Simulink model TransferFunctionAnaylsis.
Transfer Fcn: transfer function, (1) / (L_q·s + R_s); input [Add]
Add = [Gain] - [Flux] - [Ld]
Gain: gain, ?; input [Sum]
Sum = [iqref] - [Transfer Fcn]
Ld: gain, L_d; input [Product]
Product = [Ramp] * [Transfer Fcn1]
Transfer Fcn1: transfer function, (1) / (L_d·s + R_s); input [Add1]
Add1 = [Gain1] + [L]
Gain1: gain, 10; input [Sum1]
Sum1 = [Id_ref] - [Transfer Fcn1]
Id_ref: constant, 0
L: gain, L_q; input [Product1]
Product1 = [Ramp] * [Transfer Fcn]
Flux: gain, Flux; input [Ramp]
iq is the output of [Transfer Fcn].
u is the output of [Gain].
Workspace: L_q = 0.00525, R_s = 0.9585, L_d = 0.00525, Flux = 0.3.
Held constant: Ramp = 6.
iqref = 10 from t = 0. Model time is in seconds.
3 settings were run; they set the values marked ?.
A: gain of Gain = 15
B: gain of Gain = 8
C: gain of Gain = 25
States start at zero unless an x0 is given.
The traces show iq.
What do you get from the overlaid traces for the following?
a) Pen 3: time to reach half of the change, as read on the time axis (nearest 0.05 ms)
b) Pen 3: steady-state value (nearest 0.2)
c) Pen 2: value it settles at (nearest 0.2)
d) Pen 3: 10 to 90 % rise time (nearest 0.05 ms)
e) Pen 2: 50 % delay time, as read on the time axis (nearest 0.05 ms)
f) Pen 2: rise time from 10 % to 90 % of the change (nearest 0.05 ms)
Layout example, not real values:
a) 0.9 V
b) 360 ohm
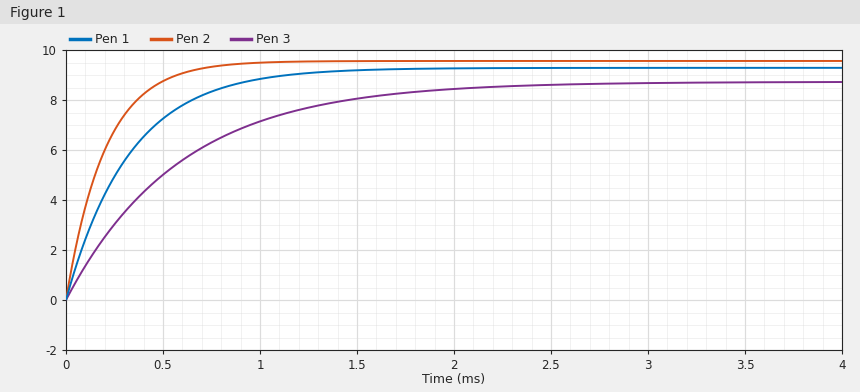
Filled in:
a) 0.40 ms
b) 8.8
c) 9.6
d) 1.30 ms
e) 0.15 ms
f) 0.45 ms
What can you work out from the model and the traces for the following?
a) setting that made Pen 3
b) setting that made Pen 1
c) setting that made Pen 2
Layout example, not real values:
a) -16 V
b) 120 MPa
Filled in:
a) B
b) A
c) C
